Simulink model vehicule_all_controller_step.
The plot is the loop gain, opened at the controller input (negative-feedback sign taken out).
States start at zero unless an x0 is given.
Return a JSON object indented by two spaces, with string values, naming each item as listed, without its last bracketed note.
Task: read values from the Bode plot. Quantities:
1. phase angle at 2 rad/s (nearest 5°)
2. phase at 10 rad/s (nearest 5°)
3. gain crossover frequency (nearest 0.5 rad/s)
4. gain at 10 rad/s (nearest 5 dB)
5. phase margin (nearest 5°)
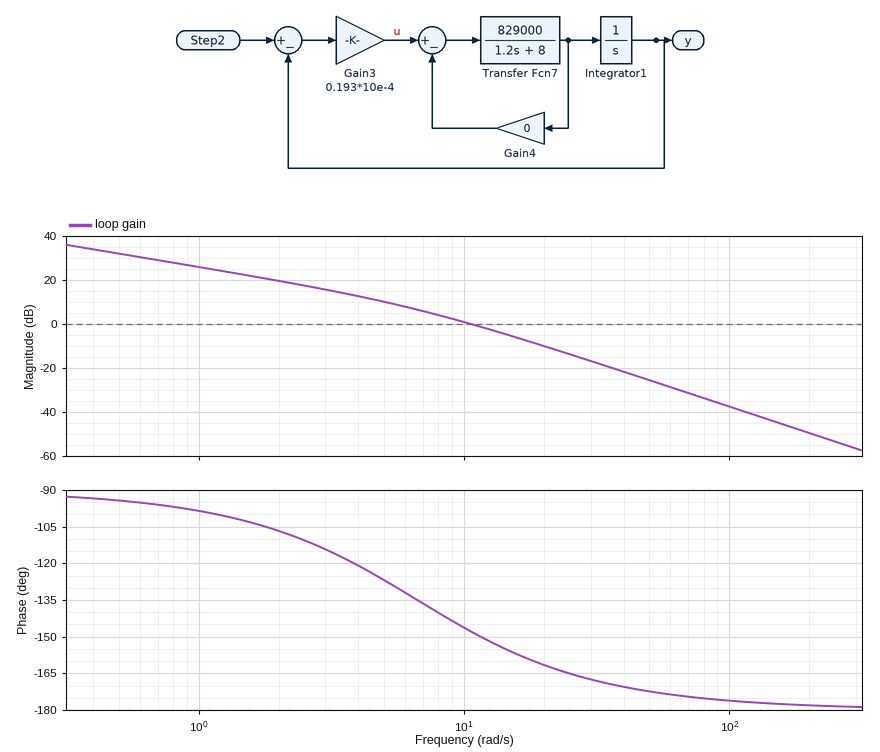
{
  "phase angle at 2 rad/s": "-105°",
  "phase at 10 rad/s": "-145°",
  "gain crossover frequency": "10.5 rad/s",
  "gain at 10 rad/s": "0 dB",
  "phase margin": "30°"
}
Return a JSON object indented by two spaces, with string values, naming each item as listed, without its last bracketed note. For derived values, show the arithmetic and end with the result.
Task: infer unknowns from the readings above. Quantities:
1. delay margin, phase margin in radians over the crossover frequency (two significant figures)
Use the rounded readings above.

{
  "delay margin, phase margin in radians over the crossover frequency": "30 × π / 180 / 10.5 = 0.050 s"
}
